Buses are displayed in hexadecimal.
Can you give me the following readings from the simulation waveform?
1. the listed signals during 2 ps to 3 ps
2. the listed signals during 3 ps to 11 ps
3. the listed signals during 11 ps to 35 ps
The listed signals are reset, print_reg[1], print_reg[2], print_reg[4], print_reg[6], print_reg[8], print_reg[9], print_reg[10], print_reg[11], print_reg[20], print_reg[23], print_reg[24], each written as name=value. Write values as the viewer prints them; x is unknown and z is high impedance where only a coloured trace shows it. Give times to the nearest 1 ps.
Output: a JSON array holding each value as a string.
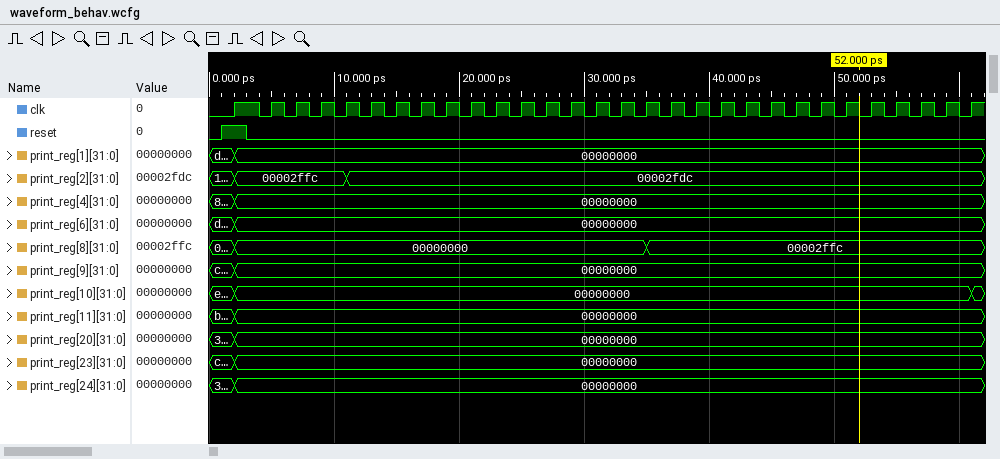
["reset=1, print_reg[1]=00000000, print_reg[2]=00002ffc, print_reg[4]=00000000, print_reg[6]=00000000, print_reg[8]=00000000, print_reg[9]=00000000, print_reg[10]=00000000, print_reg[11]=00000000, print_reg[20]=00000000, print_reg[23]=00000000, print_reg[24]=00000000", "reset=0, print_reg[1]=00000000, print_reg[2]=00002ffc, print_reg[4]=00000000, print_reg[6]=00000000, print_reg[8]=00000000, print_reg[9]=00000000, print_reg[10]=00000000, print_reg[11]=00000000, print_reg[20]=00000000, print_reg[23]=00000000, print_reg[24]=00000000", "reset=0, print_reg[1]=00000000, print_reg[2]=00002fdc, print_reg[4]=00000000, print_reg[6]=00000000, print_reg[8]=00000000, print_reg[9]=00000000, print_reg[10]=00000000, print_reg[11]=00000000, print_reg[20]=00000000, print_reg[23]=00000000, print_reg[24]=00000000"]
